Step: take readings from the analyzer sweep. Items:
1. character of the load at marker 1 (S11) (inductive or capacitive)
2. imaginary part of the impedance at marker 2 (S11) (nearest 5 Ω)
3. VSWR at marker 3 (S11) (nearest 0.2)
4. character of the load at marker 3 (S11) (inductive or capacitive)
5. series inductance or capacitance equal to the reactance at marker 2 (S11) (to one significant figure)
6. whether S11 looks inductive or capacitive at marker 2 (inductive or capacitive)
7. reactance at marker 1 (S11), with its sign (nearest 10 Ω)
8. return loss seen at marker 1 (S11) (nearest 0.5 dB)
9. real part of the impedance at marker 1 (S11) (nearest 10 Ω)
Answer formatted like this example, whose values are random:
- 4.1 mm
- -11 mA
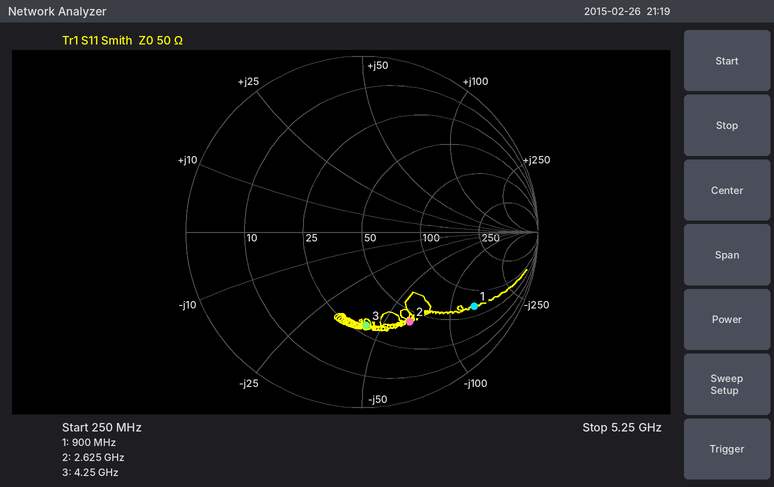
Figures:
- capacitive
- -65 Ω
- 3.2
- capacitive
- 900 fF
- capacitive
- -140 Ω
- 2.5 dB
- 70 Ω
